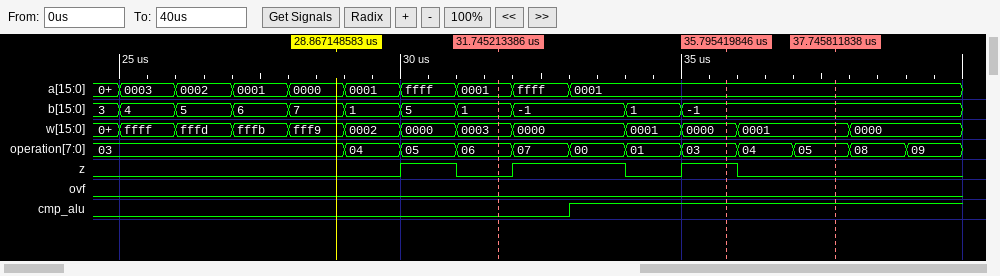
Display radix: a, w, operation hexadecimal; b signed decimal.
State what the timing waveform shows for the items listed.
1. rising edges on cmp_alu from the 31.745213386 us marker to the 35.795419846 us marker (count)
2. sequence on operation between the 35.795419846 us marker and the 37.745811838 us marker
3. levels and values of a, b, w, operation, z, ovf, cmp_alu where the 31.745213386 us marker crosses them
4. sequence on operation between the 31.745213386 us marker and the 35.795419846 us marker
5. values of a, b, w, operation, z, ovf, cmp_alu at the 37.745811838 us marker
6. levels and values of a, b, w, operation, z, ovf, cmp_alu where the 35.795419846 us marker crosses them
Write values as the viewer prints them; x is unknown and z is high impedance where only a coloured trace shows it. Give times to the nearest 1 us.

1
03, 04, 05
a=0001, b=1, w=0003, operation=06, z=0, ovf=0, cmp_alu=0
06, 07, 00, 01, 03
a=0001, b=-1, w=0001, operation=05, z=0, ovf=0, cmp_alu=1
a=0001, b=-1, w=0000, operation=03, z=1, ovf=0, cmp_alu=1
